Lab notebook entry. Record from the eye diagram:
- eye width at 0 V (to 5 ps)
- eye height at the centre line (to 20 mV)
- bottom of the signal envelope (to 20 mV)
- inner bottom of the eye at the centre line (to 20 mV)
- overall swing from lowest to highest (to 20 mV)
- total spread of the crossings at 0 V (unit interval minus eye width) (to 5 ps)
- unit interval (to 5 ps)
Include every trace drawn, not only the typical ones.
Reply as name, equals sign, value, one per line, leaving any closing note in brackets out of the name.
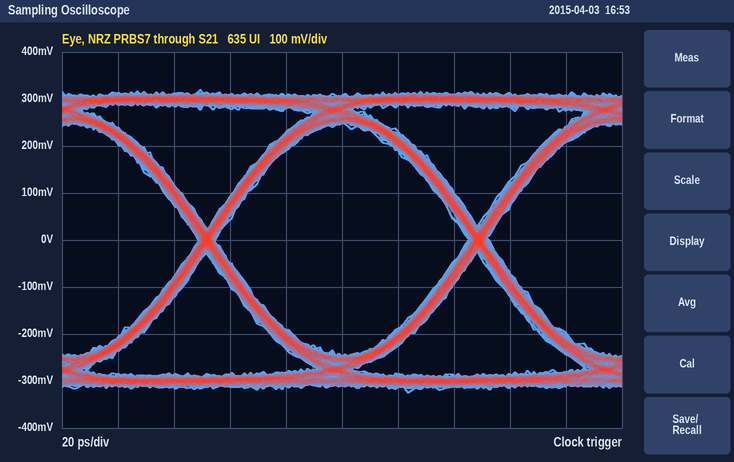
eye width at 0 V = 90 ps
eye height at the centre line = 500 mV
bottom of the signal envelope = -320 mV
inner bottom of the eye at the centre line = -240 mV
overall swing from lowest to highest = 640 mV
total spread of the crossings at 0 V (unit interval minus eye width) = 5 ps
unit interval = 95 ps
